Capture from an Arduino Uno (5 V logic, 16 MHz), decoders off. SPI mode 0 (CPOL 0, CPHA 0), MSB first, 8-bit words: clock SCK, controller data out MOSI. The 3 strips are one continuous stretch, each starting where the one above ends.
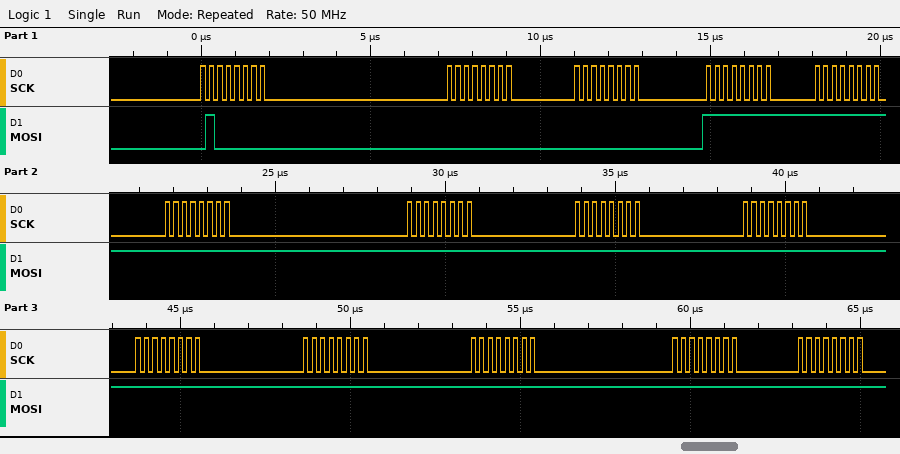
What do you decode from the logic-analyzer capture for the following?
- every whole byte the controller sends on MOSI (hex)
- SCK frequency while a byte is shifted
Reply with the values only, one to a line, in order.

40 00 00 FF FF FF FF FF FF FF FF FF FF FF
4 MHz
